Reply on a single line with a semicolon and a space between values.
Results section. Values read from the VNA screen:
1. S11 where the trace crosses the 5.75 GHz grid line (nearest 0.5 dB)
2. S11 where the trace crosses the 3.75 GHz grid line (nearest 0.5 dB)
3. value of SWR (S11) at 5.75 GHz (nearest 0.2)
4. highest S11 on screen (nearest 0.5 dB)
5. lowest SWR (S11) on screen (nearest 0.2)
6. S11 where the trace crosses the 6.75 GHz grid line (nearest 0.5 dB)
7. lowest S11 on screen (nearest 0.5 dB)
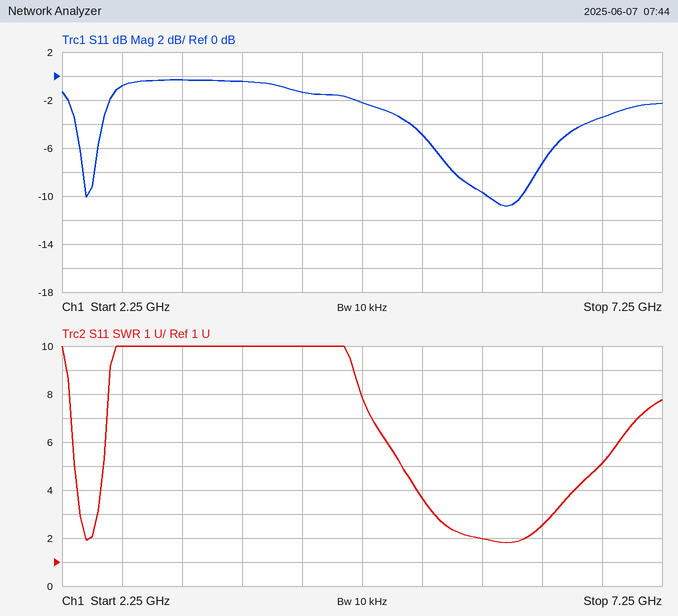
-9.5 dB; -0.5 dB; 2.0; -0.5 dB; 1.8; -3.5 dB; -11.0 dB
